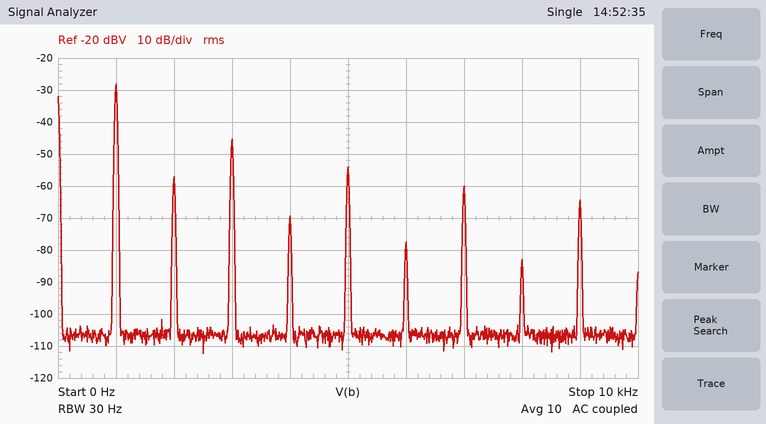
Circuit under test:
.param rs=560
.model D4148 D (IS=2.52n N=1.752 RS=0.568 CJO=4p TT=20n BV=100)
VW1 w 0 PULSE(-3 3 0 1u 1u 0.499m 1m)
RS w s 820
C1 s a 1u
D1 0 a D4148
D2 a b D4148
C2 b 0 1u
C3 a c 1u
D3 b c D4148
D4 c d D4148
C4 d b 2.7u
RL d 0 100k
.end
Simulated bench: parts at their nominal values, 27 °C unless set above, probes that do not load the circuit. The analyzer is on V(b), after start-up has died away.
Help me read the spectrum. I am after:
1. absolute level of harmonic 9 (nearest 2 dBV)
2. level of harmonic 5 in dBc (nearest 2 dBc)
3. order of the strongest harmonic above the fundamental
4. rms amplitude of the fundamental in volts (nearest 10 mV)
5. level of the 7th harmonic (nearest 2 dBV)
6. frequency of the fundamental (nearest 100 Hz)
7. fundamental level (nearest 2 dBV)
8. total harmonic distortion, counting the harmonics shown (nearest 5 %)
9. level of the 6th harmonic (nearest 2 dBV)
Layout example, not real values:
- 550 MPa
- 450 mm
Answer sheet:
- -64 dBV
- -26 dBc
- 3
- 40 mV
- -60 dBV
- 1.0 kHz
- -28 dBV
- 15 %
- -78 dBV
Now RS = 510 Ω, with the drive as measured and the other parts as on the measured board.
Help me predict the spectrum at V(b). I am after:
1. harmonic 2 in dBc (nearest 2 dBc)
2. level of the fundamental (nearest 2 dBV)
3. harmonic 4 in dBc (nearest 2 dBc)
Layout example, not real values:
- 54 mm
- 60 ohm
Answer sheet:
- -30 dBc
- -28 dBV
- -44 dBc
